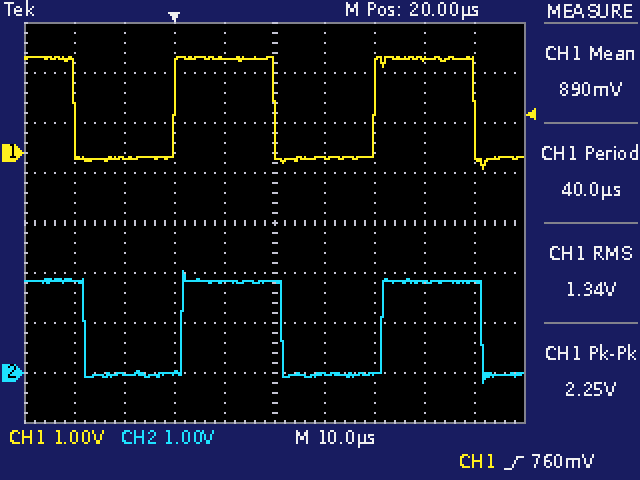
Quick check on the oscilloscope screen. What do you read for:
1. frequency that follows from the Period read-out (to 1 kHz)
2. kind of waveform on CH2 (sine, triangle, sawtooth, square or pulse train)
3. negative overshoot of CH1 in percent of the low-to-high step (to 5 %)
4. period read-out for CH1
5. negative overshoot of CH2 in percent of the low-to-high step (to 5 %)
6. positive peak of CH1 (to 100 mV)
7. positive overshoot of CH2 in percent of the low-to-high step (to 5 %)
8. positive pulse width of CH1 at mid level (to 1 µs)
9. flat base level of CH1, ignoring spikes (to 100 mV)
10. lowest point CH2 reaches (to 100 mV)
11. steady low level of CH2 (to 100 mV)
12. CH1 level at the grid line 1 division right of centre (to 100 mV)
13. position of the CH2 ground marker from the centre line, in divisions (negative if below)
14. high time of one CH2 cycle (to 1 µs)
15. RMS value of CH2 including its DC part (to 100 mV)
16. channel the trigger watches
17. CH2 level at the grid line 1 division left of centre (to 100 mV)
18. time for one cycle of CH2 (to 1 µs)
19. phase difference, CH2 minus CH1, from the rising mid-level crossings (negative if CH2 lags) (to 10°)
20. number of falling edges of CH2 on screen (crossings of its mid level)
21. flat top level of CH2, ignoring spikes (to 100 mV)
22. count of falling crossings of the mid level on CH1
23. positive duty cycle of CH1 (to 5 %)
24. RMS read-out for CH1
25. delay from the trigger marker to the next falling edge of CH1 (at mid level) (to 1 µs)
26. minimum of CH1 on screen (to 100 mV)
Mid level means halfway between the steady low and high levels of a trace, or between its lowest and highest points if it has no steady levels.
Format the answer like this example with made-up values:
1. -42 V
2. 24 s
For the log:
1. 25 kHz
2. square
3. 10 %
4. 40.0 µs
5. 10 %
6. 1.9 V
7. 10 %
8. 20 µs
9. -100 mV
10. -200 mV
11. 0.0 V
12. -100 mV
13. -3.0 div
14. 20 µs
15. 1.3 V
16. CH1
17. 1.8 V
18. 40 µs
19. -10°
20. 3
21. 1.8 V
22. 3
23. 50 %
24. 1.34 V
25. 20 µs
26. -300 mV
